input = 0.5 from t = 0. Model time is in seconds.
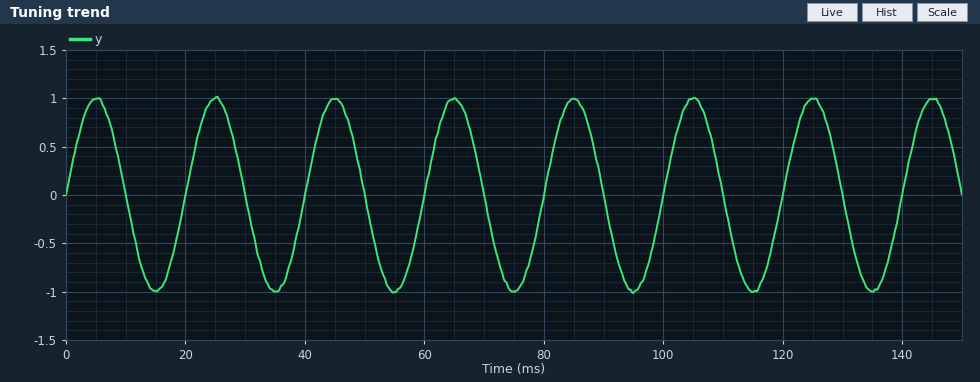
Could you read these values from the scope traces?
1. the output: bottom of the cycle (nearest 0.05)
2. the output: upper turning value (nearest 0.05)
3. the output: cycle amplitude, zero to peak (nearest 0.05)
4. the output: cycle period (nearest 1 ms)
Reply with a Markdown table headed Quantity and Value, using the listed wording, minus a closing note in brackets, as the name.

| Quantity | Value |
|---|---|
| the output: bottom of the cycle | -1.00 |
| the output: upper turning value | 1.00 |
| the output: cycle amplitude, zero to peak | 1.00 |
| the output: cycle period | 20 ms |
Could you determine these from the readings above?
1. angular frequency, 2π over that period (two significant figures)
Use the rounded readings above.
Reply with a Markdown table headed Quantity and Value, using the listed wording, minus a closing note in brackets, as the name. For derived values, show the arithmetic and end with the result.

| Quantity | Value |
|---|---|
| angular frequency, 2π over that period | 2π / 20 = 0.31 rad/ms |
